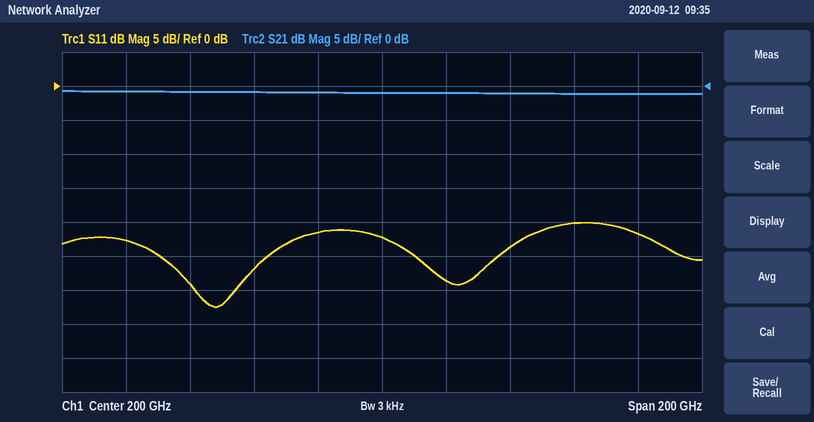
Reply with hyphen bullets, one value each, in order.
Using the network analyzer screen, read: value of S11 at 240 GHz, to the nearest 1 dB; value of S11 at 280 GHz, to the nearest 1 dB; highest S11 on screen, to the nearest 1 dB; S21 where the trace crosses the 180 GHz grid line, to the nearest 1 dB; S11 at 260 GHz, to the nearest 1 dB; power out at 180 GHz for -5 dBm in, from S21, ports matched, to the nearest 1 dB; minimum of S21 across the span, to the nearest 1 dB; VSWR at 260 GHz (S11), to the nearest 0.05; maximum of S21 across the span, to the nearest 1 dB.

- -24 dB
- -22 dB
- -20 dB
- -1 dB
- -20 dB
- -6 dBm
- -1 dB
- 1.20
- -1 dB
